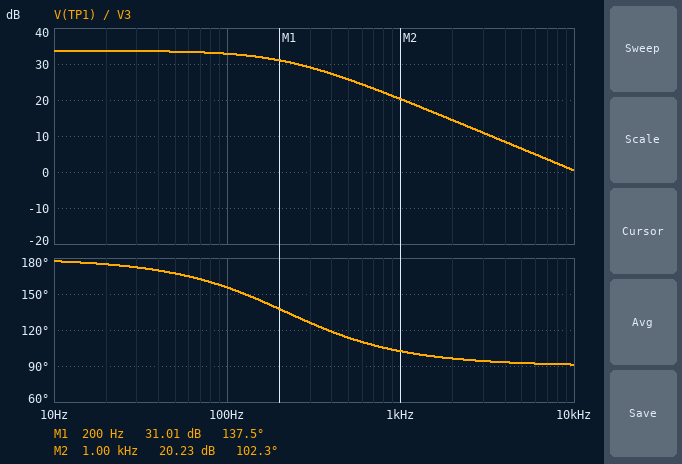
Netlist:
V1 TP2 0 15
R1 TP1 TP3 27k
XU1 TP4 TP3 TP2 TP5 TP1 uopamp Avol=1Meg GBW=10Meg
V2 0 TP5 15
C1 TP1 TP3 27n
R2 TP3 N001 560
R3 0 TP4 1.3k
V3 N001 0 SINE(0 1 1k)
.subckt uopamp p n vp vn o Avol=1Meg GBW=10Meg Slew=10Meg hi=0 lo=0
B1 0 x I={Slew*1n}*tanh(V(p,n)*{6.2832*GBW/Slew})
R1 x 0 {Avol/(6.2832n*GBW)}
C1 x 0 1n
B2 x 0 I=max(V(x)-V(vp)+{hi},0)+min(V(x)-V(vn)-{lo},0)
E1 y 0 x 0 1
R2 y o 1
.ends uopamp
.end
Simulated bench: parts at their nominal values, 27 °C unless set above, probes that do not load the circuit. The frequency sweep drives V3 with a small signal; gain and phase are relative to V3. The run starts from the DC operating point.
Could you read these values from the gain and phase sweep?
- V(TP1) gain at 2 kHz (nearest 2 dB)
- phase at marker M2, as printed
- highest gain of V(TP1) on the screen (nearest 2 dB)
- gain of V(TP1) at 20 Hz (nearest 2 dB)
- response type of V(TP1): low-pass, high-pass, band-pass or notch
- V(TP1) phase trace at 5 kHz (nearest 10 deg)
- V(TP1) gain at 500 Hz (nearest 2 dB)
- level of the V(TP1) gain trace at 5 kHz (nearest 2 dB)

14 dB
102.3 deg
34 dB
34 dB
low-pass
90 deg
26 dB
6 dB
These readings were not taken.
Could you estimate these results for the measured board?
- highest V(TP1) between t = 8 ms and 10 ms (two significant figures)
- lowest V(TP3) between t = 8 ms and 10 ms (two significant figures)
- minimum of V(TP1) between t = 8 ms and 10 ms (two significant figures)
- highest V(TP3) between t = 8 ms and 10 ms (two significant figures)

10 V
-1.0 mV
-10 V
1.0 mV
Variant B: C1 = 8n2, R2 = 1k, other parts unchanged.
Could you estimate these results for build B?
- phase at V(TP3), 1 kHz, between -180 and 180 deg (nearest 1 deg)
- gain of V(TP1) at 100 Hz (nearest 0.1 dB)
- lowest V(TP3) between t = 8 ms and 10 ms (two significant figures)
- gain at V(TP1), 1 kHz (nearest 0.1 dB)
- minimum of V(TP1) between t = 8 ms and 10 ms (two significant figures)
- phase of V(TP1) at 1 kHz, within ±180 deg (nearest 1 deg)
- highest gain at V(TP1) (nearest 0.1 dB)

35 deg
28.5 dB
-180 mV
23.9 dB
-15 V
126 deg
28.6 dB
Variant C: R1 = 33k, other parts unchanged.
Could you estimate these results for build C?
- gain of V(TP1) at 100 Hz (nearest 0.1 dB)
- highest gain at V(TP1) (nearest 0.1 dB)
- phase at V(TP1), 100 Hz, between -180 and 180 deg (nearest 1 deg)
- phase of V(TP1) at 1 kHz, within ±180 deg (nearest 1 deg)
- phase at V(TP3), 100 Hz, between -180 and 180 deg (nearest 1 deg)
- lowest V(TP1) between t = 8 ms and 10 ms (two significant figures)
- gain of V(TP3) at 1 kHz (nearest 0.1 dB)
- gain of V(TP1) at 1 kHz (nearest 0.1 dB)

34.2 dB
35.4 dB
151 deg
100 deg
55 deg
-10 V
-59.7 dB
20.3 dB
